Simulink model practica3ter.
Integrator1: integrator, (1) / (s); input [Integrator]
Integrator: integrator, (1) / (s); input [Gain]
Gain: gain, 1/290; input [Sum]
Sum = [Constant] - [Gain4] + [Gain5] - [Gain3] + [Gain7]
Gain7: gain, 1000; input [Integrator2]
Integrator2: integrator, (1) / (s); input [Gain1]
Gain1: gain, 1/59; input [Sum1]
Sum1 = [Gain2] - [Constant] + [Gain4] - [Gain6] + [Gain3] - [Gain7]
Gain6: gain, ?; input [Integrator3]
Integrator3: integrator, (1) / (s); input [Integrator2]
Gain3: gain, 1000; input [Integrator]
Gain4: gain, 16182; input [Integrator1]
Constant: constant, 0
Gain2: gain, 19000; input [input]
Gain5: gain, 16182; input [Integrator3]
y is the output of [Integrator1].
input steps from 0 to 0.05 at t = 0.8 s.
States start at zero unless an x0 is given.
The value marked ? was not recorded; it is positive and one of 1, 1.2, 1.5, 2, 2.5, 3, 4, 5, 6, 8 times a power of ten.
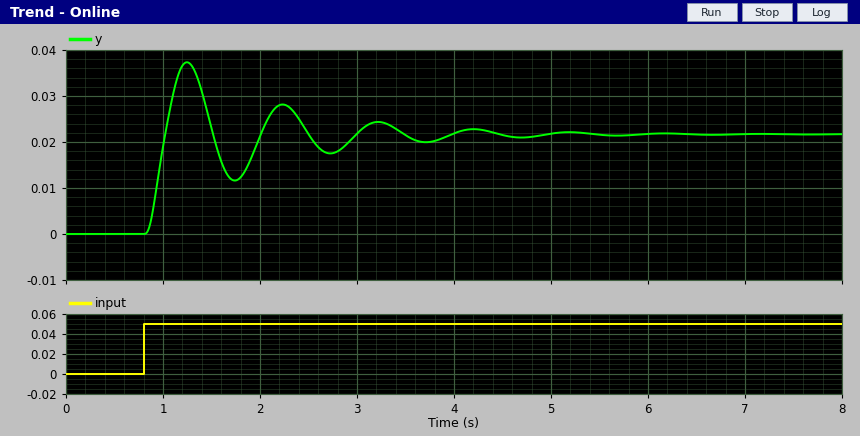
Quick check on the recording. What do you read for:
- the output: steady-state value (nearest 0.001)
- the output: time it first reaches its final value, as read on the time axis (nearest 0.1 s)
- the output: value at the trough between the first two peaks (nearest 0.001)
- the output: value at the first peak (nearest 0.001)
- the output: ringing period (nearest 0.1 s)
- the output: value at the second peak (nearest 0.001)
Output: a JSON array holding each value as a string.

["0.022", "1.0 s", "0.012", "0.037", "1.0 s", "0.028"]
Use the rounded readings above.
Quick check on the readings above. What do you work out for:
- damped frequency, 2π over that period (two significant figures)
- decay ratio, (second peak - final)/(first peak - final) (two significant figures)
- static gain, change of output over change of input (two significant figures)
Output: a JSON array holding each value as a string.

["6.3 rad/s", "0.40", "0.44"]
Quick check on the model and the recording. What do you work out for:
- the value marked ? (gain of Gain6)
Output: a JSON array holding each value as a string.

["60000"]
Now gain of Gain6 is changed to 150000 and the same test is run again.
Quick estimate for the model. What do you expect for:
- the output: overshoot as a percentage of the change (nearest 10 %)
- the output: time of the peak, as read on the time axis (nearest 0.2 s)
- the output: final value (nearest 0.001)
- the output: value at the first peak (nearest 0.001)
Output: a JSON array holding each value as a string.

["60 %", "1.2 s", "0.007", "0.011"]
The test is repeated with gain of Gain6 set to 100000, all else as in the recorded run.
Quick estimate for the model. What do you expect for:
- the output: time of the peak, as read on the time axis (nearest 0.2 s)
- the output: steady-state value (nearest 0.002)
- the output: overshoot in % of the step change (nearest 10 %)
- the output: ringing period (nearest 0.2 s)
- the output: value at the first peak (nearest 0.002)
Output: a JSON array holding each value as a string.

["1.2 s", "0.012", "60 %", "1.0 s", "0.018"]
